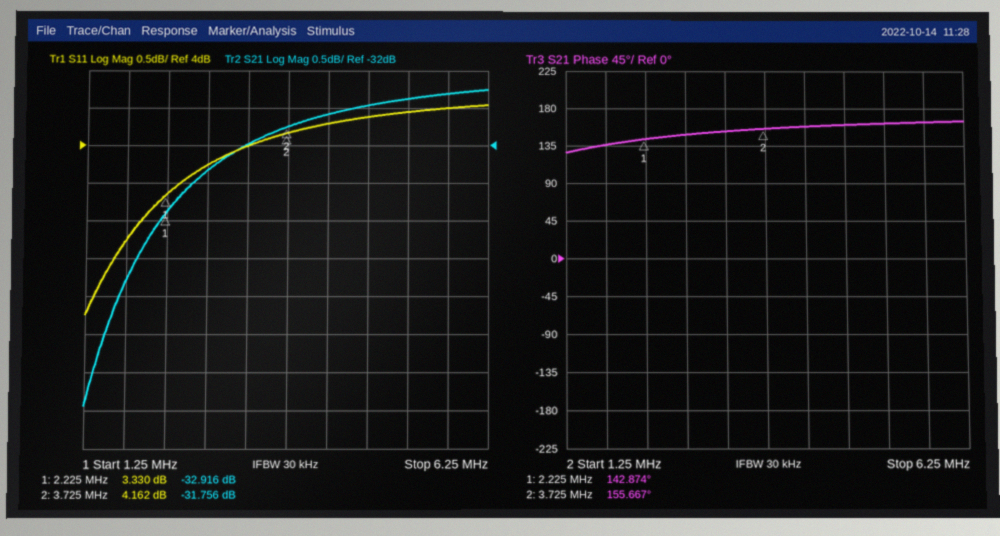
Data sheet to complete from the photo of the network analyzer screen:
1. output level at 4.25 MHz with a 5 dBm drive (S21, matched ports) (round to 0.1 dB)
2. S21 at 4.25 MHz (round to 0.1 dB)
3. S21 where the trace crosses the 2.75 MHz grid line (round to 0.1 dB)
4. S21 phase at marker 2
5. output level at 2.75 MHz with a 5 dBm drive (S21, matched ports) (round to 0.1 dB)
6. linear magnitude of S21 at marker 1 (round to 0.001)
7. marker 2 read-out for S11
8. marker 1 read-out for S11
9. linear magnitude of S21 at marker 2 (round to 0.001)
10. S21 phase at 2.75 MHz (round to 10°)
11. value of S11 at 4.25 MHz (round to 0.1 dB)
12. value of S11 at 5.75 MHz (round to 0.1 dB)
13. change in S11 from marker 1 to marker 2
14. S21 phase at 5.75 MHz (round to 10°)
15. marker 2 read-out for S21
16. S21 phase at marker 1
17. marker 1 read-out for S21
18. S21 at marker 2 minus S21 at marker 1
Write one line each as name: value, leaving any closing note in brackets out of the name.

output level at 4.25 MHz with a 5 dBm drive (S21, matched ports): -26.6 dBm
S21 at 4.25 MHz: -31.6 dB
S21 where the trace crosses the 2.75 MHz grid line: -32.3 dB
S21 phase at marker 2: 155.667°
output level at 2.75 MHz with a 5 dBm drive (S21, matched ports): -27.3 dBm
linear magnitude of S21 at marker 1: 0.023
marker 2 read-out for S11: 4.162 dB
marker 1 read-out for S11: 3.330 dB
linear magnitude of S21 at marker 2: 0.026
S21 phase at 2.75 MHz: 150°
value of S11 at 4.25 MHz: 4.3 dB
value of S11 at 5.75 MHz: 4.5 dB
change in S11 from marker 1 to marker 2: 0.832 dB
S21 phase at 5.75 MHz: 160°
marker 2 read-out for S21: -31.756 dB
S21 phase at marker 1: 142.874°
marker 1 read-out for S21: -32.916 dB
S21 at marker 2 minus S21 at marker 1: 1.160 dB
